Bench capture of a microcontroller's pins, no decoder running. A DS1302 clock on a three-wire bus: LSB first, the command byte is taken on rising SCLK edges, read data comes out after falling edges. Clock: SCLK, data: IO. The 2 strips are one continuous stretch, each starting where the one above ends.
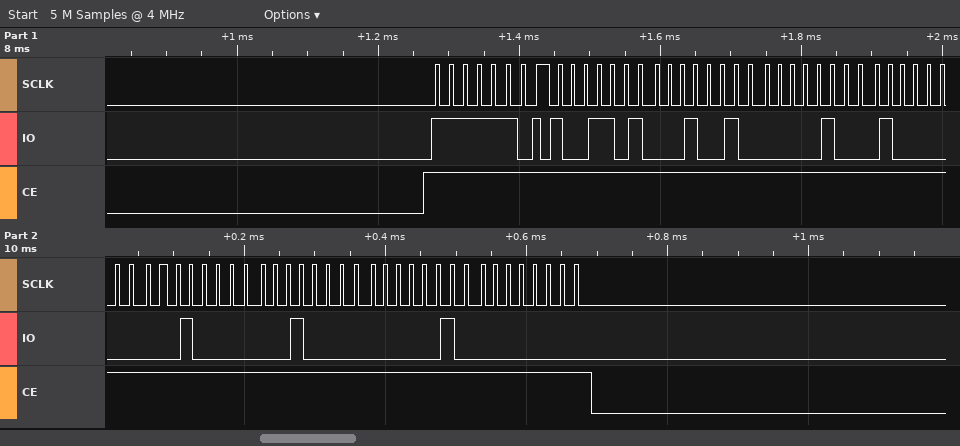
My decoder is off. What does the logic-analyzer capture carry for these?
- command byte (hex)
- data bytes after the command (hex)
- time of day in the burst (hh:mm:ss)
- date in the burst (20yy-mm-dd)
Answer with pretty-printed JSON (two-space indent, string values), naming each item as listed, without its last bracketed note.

{
  "command byte": "0xBF",
  "data bytes after the command": "59 24 10 01 04 04 20 00",
  "time of day in the burst": "10:24:59",
  "date in the burst": "2020-04-01"
}
